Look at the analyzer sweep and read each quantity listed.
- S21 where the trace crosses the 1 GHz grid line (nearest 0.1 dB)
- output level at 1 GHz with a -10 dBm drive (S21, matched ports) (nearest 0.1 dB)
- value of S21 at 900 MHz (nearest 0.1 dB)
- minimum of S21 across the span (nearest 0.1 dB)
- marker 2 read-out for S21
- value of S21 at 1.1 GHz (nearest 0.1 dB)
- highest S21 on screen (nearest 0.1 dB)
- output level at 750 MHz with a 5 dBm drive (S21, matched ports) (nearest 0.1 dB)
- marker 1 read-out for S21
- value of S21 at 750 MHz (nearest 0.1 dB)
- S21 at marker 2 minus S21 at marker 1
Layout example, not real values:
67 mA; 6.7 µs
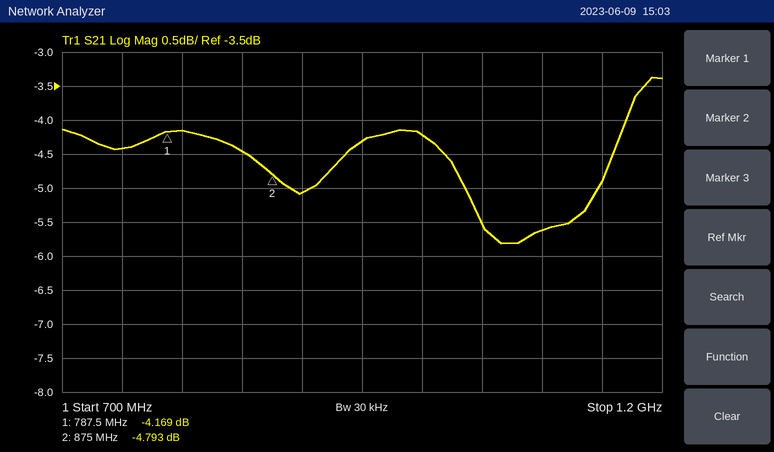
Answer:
-4.2 dB; -14.2 dBm; -5.1 dB; -5.8 dB; -4.793 dB; -5.6 dB; -3.4 dB; 0.6 dBm; -4.169 dB; -4.4 dB; -0.624 dB
